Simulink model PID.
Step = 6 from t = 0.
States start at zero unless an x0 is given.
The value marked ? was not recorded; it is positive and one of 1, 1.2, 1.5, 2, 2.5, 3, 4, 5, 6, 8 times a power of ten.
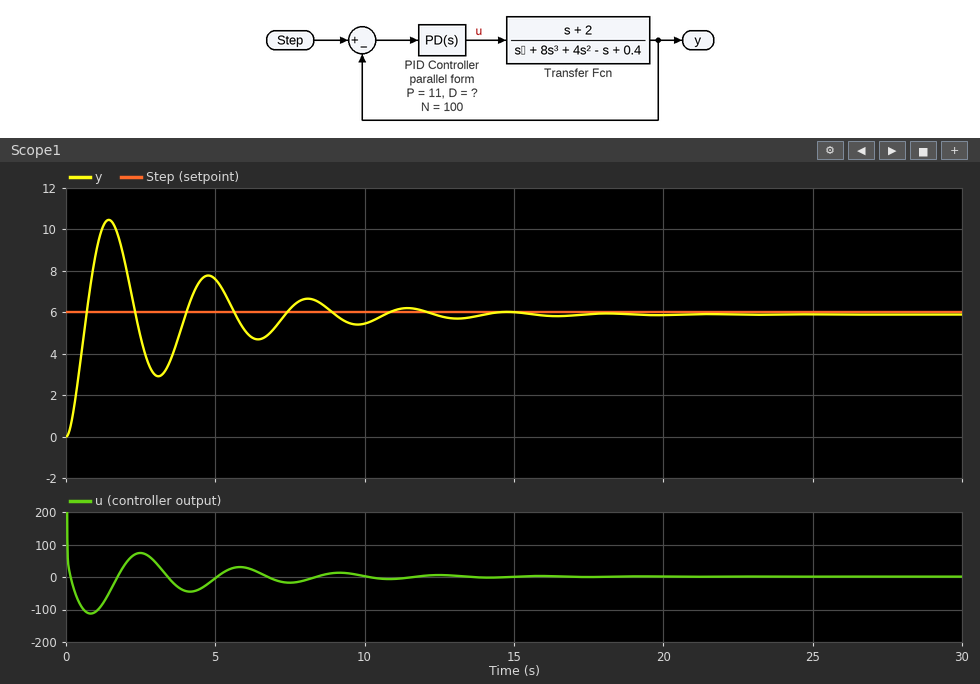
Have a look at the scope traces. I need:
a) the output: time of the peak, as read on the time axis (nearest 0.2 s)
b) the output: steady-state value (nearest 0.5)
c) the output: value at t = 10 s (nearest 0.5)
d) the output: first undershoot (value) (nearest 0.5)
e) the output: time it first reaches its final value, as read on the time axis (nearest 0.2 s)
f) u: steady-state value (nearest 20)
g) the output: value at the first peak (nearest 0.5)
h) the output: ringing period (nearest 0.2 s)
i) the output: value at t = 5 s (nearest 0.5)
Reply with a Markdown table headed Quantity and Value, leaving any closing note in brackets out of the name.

| Quantity | Value |
|---|---|
| the output: time of the peak, as read on the time axis | 1.4 s |
| the output: steady-state value | 6.0 |
| the output: value at t = 10 s | 5.5 |
| the output: first undershoot (value) | 3.0 |
| the output: time it first reaches its final value, as read on the time axis | 0.6 s |
| u: steady-state value | 0 |
| the output: value at the first peak | 10.5 |
| the output: ringing period | 3.4 s |
| the output: value at t = 5 s | 7.5 |
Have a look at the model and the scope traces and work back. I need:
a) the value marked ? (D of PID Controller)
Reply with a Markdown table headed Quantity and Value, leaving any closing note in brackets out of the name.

| Quantity | Value |
|---|---|
| the value marked ? | 10 |
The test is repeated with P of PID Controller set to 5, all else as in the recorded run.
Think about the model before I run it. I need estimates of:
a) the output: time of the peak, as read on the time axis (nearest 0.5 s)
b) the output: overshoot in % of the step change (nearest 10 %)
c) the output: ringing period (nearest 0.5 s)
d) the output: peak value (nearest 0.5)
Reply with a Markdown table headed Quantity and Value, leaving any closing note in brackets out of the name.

| Quantity | Value |
|---|---|
| the output: time of the peak, as read on the time axis | 1.5 s |
| the output: overshoot in % of the step change | 60 % |
| the output: ringing period | 4.0 s |
| the output: peak value | 9.5 |
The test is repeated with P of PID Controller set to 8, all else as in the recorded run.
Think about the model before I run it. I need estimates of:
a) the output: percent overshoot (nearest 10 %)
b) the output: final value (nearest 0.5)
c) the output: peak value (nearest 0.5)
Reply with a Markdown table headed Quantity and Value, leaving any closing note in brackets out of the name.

| Quantity | Value |
|---|---|
| the output: percent overshoot | 70 % |
| the output: final value | 6.0 |
| the output: peak value | 10.0 |
